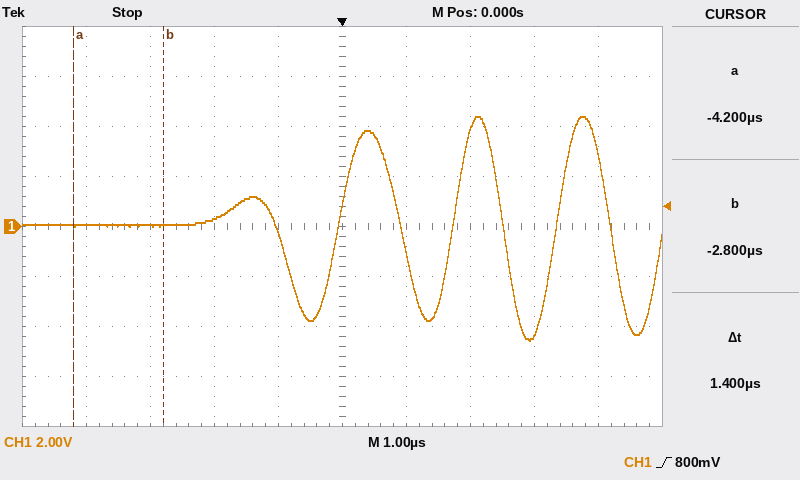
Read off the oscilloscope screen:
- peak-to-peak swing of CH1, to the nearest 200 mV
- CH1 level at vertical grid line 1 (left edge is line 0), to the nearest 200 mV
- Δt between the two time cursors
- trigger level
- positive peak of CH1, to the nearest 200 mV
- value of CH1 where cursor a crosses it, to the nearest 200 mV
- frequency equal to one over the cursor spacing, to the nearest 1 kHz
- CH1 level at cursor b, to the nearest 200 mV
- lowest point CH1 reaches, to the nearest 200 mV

9.0 V
0.0 V
1.4 µs
800 mV
4.4 V
0.0 V
714 kHz
0.0 V
-4.6 V
